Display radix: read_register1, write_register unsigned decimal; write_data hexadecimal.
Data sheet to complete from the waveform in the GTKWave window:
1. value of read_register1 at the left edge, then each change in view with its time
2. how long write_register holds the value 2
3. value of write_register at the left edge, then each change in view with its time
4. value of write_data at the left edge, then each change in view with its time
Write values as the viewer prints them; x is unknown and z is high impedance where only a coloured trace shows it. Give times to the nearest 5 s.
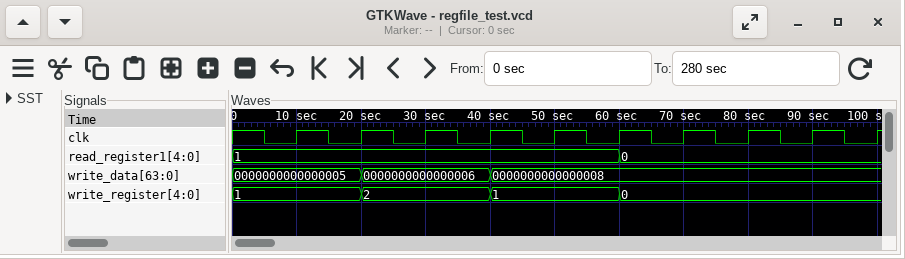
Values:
1, 0 at 60 s
20 s
1, 2 at 20 s, 1 at 40 s, 0 at 60 s
0000000000000005, 0000000000000006 at 20 s, 0000000000000008 at 40 s
